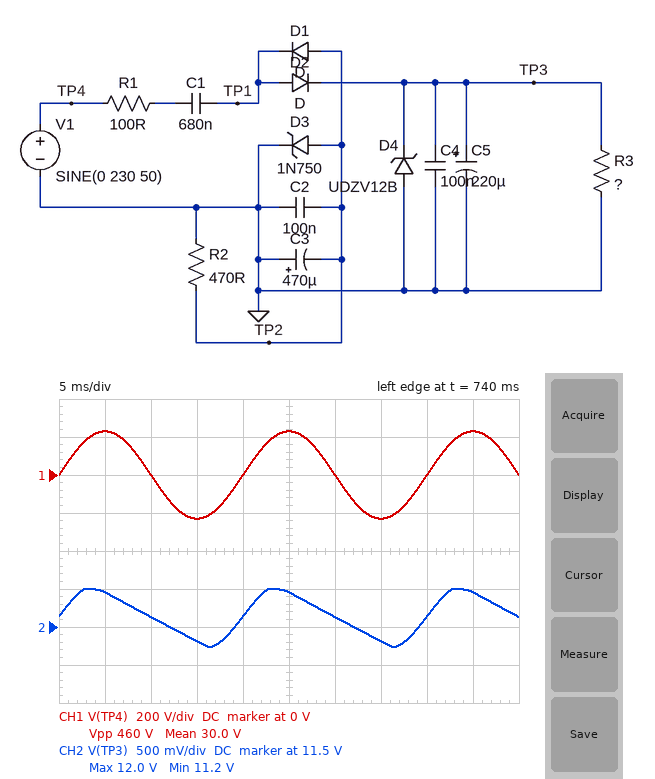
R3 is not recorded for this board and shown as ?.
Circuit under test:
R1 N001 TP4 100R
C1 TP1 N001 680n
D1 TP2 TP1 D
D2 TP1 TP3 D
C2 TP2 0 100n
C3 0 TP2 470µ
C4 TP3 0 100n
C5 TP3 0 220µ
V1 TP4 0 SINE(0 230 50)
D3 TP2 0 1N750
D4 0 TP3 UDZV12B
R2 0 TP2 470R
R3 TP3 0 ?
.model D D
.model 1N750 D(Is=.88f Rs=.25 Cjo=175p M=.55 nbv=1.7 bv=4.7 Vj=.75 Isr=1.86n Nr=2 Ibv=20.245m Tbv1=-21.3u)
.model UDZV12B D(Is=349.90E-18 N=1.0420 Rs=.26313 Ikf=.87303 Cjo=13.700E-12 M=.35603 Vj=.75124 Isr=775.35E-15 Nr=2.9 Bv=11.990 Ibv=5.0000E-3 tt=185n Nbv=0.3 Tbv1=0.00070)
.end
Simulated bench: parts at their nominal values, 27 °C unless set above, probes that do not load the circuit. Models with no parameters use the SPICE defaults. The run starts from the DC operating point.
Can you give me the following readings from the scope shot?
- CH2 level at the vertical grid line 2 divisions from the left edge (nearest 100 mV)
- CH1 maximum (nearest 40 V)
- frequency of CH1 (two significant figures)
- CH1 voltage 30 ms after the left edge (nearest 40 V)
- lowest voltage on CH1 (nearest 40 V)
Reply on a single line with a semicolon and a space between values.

11.6 V; 240 V; 50 Hz; 0 V; -240 V
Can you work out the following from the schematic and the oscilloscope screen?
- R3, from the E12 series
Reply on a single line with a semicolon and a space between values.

820 Ω
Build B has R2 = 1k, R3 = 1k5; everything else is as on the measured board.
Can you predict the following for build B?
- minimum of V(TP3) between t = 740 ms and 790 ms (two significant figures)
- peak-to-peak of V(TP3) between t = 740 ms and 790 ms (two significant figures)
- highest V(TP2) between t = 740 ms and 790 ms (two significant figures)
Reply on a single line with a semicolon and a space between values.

12 V; 440 mV; -4.5 V
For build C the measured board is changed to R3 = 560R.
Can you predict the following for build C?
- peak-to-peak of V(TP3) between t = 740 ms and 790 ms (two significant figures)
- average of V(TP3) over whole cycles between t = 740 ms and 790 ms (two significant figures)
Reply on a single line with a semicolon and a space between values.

800 mV; 8.5 V
